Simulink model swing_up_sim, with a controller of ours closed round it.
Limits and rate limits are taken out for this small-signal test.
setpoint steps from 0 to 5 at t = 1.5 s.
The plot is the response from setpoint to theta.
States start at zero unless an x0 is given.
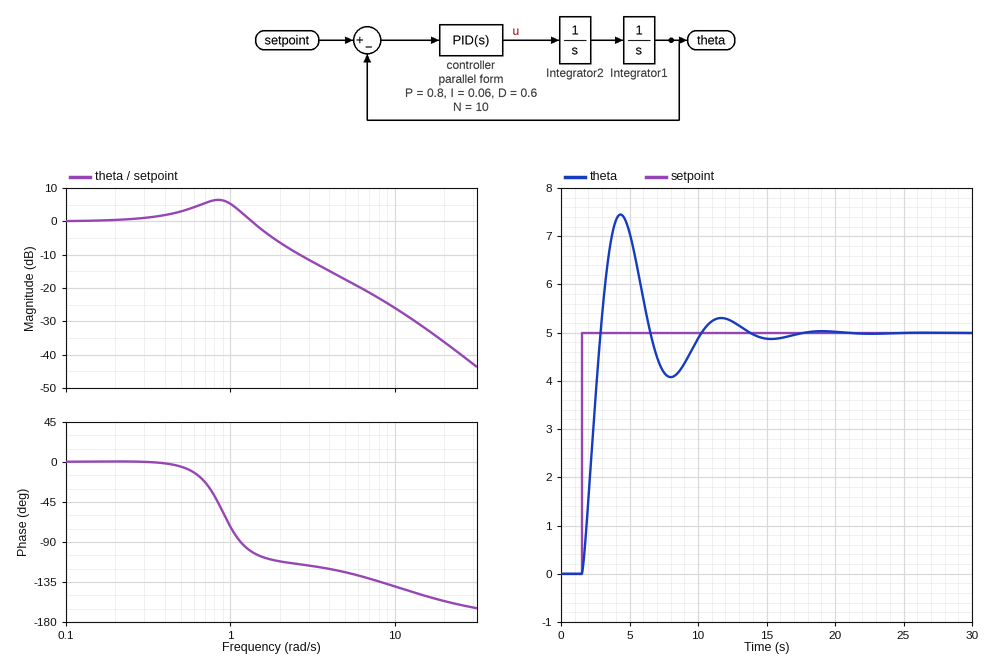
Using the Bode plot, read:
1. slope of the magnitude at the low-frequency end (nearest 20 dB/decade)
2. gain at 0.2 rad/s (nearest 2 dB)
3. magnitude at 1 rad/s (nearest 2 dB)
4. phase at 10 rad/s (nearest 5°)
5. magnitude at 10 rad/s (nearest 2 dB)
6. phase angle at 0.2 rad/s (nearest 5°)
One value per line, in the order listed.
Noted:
0 dB/decade
0 dB
6 dB
-140°
-26 dB
0°
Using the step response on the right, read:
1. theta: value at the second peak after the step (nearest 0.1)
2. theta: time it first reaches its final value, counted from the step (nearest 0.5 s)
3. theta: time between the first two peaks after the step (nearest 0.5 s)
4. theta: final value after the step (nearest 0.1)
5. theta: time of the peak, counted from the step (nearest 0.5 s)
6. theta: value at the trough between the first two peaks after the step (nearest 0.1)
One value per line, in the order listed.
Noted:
5.3
1.5 s
7.5 s
5.0
3.0 s
4.1
